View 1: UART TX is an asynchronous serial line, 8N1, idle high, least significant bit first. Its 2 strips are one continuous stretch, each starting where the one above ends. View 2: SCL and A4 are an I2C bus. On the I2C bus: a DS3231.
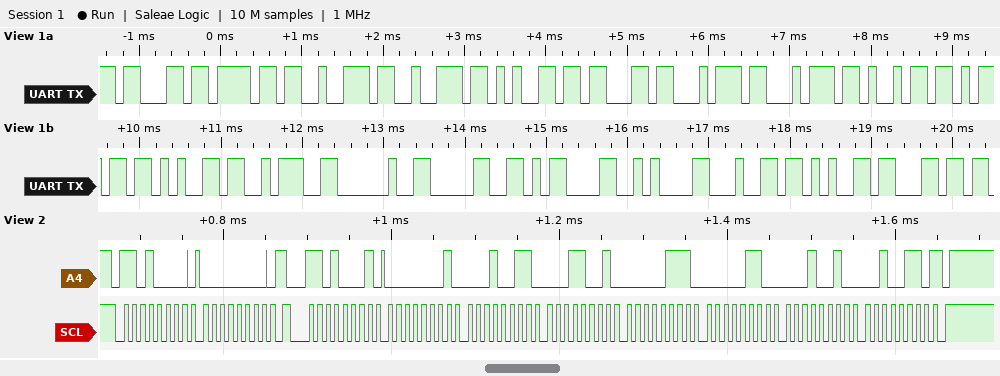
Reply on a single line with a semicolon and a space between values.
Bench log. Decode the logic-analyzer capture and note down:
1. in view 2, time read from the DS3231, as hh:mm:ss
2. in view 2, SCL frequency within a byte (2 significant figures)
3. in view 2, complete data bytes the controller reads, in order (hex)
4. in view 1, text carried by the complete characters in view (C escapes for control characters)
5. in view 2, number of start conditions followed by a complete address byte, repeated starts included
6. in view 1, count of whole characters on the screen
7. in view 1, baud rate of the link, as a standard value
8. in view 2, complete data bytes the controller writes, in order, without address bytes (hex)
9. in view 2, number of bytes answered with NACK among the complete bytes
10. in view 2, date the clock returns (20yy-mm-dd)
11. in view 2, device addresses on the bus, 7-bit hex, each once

19:13:01; 100 kHz; 01 13 19 07 06 12 26; "correcttime: 0\r\ndel"; 2; 19; 9600 baud; 00; 1; 2026-12-06; 0x68
